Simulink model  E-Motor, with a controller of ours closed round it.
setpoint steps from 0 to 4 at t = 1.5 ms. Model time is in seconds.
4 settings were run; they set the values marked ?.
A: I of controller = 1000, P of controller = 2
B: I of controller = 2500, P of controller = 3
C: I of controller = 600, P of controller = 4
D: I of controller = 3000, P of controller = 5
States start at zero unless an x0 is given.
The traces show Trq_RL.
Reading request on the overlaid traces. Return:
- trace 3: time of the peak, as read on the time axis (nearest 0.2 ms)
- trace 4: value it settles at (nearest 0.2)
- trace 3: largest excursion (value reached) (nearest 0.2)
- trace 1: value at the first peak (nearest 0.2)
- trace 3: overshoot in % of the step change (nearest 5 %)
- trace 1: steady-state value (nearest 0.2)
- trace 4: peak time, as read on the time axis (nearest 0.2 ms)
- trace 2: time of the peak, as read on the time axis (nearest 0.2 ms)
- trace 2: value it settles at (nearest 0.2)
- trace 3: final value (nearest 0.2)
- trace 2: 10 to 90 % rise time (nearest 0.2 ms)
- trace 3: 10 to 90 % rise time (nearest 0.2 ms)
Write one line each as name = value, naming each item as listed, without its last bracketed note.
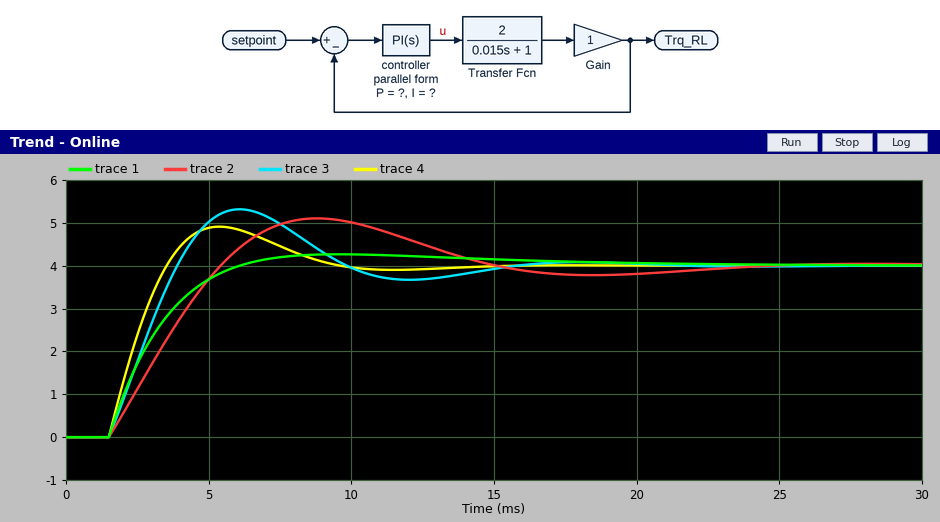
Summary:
trace 3: time of the peak, as read on the time axis = 6.0 ms
trace 4: value it settles at = 4.0
trace 3: largest excursion (value reached) = 5.4
trace 1: value at the first peak = 4.2
trace 3: overshoot in % of the step change = 35 %
trace 1: steady-state value = 4.0
trace 4: peak time, as read on the time axis = 5.4 ms
trace 2: time of the peak, as read on the time axis = 8.8 ms
trace 2: value it settles at = 4.0
trace 3: final value = 4.0
trace 2: 10 to 90 % rise time = 3.0 ms
trace 3: 10 to 90 % rise time = 1.8 ms
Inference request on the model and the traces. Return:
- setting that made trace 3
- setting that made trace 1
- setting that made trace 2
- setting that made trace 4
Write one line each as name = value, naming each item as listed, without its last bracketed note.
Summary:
setting that made trace 3 = B
setting that made trace 1 = C
setting that made trace 2 = A
setting that made trace 4 = D
